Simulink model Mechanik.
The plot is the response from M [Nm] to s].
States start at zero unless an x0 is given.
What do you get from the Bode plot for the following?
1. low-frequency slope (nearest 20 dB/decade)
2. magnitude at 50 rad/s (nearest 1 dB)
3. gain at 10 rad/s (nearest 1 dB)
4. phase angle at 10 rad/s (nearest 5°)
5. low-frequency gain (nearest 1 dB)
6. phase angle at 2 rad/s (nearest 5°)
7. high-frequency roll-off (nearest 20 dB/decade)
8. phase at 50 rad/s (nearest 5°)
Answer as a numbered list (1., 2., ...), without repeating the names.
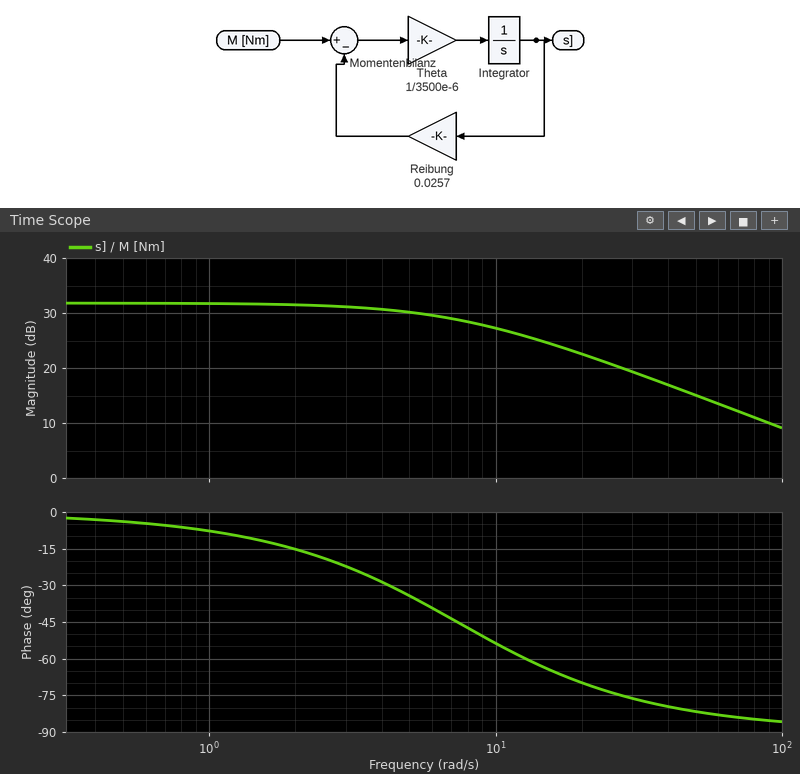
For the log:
1. 0 dB/decade
2. 15 dB
3. 27 dB
4. -55°
5. 32 dB
6. -15°
7. -20 dB/decade
8. -80°
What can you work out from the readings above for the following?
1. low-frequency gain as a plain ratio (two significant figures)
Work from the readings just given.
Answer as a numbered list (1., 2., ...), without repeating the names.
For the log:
1. 40
